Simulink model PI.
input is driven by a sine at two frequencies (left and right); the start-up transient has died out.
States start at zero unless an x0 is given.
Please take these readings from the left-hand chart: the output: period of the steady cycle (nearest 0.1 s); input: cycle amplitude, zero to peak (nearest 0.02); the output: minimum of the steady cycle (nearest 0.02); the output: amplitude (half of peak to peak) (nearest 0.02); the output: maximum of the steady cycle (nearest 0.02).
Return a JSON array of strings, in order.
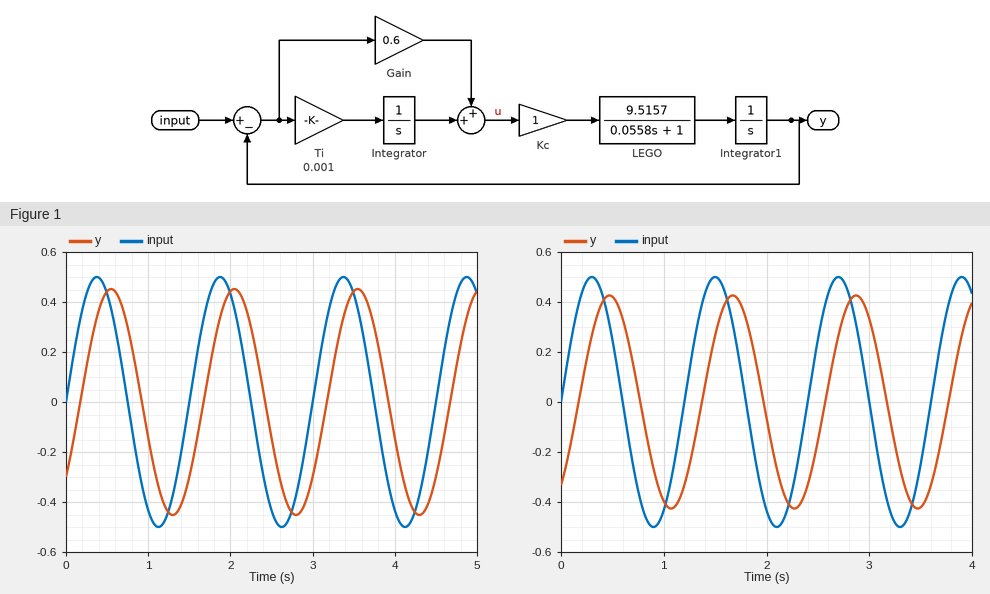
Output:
["1.5 s", "0.50", "-0.46", "0.46", "0.46"]
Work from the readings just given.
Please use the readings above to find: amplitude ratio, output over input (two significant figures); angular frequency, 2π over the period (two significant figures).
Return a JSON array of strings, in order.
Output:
["0.92", "4.2 rad/s"]
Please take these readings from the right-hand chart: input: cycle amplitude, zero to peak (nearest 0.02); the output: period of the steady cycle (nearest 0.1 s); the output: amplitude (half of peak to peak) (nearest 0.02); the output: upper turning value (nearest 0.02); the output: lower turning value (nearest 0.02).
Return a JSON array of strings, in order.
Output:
["0.50", "1.2 s", "0.42", "0.42", "-0.42"]
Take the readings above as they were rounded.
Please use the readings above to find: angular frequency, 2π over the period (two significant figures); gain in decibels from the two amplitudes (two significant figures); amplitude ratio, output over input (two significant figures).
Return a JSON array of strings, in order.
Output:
["5.2 rad/s", "-1.5 dB", "0.84"]
